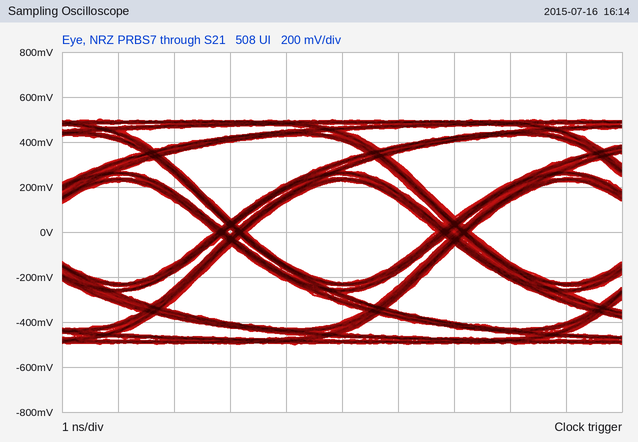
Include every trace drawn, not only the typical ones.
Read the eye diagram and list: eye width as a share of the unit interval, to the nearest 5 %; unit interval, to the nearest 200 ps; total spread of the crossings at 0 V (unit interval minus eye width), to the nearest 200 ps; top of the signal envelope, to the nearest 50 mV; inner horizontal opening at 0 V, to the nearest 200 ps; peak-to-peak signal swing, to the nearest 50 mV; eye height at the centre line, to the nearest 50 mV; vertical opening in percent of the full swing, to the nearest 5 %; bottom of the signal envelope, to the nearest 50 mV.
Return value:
85 %
4.0 ns
600 ps
500 mV
3.4 ns
1.00 V
450 mV
45 %
-500 mV
